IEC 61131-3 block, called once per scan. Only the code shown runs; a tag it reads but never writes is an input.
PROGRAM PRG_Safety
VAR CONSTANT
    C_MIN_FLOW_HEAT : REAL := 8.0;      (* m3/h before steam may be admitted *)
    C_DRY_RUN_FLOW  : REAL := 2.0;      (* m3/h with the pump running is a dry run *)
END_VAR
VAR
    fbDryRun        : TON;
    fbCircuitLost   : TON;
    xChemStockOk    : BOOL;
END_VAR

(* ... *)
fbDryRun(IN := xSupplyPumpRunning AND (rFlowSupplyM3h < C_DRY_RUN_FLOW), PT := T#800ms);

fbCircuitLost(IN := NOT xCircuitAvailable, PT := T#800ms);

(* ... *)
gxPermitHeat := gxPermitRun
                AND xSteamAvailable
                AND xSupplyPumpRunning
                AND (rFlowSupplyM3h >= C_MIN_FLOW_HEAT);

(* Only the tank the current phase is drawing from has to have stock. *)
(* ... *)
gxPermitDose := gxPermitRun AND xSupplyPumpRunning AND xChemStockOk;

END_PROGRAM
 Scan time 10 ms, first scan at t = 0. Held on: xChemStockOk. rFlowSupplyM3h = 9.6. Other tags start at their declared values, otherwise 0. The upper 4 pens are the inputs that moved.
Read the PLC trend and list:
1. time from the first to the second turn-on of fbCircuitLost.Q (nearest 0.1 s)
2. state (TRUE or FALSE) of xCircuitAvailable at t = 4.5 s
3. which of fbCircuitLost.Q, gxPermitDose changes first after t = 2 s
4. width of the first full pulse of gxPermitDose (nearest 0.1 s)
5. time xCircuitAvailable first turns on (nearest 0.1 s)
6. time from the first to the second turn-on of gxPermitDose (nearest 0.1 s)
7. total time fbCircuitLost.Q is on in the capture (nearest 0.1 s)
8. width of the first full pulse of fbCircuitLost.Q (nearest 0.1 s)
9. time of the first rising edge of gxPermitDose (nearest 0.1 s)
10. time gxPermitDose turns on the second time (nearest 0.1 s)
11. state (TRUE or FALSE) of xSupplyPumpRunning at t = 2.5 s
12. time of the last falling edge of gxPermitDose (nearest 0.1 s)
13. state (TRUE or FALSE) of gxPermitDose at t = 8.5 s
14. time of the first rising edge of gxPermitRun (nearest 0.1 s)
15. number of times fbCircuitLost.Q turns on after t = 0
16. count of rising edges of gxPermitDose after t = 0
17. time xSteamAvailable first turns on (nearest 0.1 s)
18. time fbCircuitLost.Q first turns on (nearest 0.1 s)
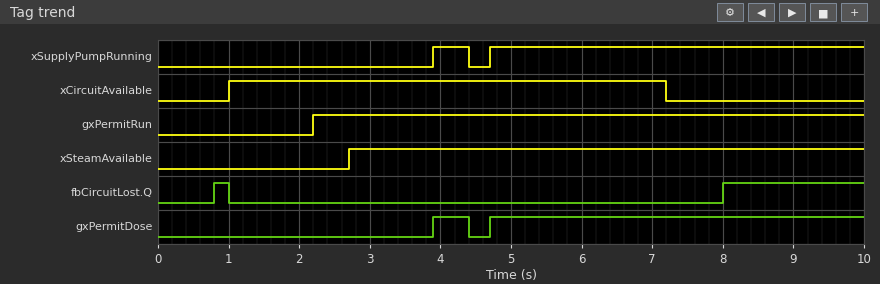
7.2 s
TRUE
gxPermitDose
0.5 s
1.0 s
0.8 s
2.2 s
0.2 s
3.9 s
4.7 s
FALSE
4.4 s
TRUE
2.2 s
2
2
2.7 s
0.8 s
